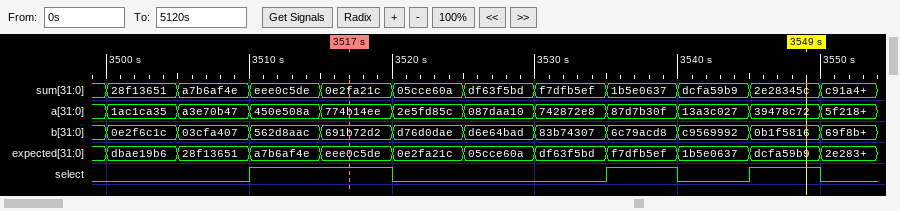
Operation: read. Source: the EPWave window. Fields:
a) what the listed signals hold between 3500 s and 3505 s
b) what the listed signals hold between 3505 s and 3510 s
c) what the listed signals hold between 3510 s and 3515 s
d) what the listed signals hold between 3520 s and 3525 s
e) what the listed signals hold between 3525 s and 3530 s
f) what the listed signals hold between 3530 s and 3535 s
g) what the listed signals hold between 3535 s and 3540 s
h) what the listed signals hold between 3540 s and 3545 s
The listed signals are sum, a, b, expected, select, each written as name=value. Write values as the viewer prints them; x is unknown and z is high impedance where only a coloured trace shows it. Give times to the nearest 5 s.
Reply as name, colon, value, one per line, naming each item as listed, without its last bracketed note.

what the listed signals hold between 3500 s and 3505 s: sum=28f13651, a=1ac1ca35, b=0e2f6c1c, expected=dbae19b6, select=0
what the listed signals hold between 3505 s and 3510 s: sum=a7b6af4e, a=a3e70b47, b=03cfa407, expected=28f13651, select=0
what the listed signals hold between 3510 s and 3515 s: sum=eee0c5de, a=450e508a, b=562d8aac, expected=a7b6af4e, select=1
what the listed signals hold between 3520 s and 3525 s: sum=05cce60a, a=2e5fd85c, b=d76d0dae, expected=0e2fa21c, select=0
what the listed signals hold between 3525 s and 3530 s: sum=df63f5bd, a=087daa10, b=d6e64bad, expected=05cce60a, select=0
what the listed signals hold between 3530 s and 3535 s: sum=f7dfb5ef, a=742872e8, b=83b74307, expected=df63f5bd, select=0
what the listed signals hold between 3535 s and 3540 s: sum=1b5e0637, a=87d7b30f, b=6c79acd8, expected=f7dfb5ef, select=1
what the listed signals hold between 3540 s and 3545 s: sum=dcfa59b9, a=13a3c027, b=c9569992, expected=1b5e0637, select=0
